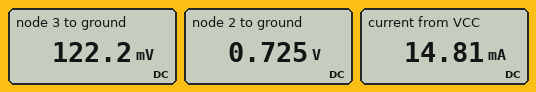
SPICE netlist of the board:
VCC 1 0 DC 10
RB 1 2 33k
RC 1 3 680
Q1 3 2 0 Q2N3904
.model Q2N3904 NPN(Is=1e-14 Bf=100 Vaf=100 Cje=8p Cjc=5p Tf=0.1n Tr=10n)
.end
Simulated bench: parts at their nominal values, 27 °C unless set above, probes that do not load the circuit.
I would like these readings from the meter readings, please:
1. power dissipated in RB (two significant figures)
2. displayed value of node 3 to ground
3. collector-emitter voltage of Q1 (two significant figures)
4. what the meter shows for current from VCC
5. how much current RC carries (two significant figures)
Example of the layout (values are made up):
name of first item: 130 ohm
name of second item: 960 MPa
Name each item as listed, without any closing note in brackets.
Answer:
power dissipated in RB: 2.6 mW
displayed value of node 3 to ground: 122.2 mV
collector-emitter voltage of Q1: 120 mV
what the meter shows for current from VCC: 14.81 mA
how much current RC carries: 15 mA
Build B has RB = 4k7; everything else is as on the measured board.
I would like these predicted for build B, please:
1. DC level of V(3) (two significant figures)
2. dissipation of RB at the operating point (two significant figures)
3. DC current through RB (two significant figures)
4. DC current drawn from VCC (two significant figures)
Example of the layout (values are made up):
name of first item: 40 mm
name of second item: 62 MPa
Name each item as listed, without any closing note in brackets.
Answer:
DC level of V(3): 60 mV
dissipation of RB at the operating point: 18 mW
DC current through RB: 2.0 mA
DC current drawn from VCC: 17 mA
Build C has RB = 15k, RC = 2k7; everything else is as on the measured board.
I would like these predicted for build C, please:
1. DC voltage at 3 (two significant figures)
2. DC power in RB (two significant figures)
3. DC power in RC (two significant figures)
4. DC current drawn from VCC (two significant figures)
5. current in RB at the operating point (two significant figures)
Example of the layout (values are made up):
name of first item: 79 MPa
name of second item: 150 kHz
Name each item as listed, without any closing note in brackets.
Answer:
DC voltage at 3: 55 mV
DC power in RB: 5.8 mW
DC power in RC: 37 mW
DC current drawn from VCC: 4.3 mA
current in RB at the operating point: 620 µA
